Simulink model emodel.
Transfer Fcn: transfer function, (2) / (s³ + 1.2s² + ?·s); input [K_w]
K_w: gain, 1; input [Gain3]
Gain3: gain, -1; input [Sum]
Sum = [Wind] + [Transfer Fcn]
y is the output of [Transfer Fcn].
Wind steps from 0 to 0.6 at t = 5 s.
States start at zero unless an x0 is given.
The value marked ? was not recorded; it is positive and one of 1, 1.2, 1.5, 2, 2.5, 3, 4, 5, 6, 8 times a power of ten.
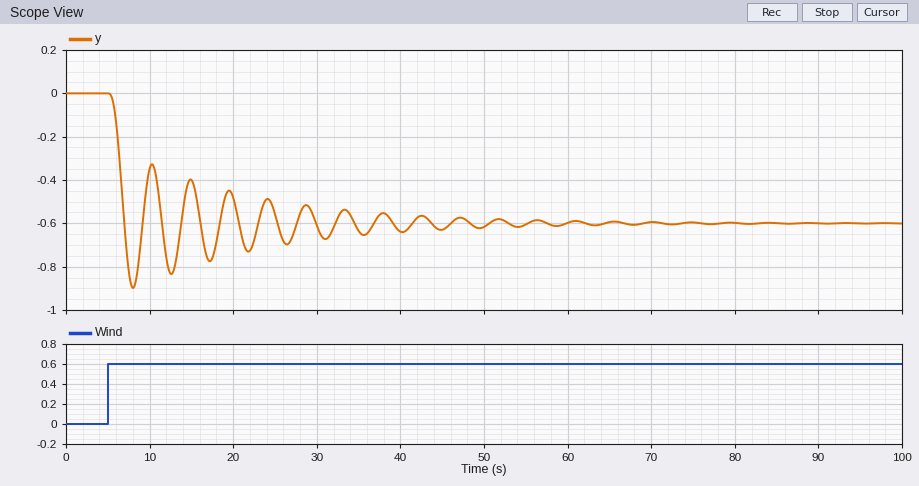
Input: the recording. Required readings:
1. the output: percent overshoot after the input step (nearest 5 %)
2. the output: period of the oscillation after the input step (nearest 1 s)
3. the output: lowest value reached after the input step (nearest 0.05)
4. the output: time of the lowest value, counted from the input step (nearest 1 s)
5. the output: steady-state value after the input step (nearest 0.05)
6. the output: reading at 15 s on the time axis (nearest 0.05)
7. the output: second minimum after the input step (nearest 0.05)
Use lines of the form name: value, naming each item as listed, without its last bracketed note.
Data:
the output: percent overshoot after the input step: 50 %
the output: period of the oscillation after the input step: 5 s
the output: lowest value reached after the input step: -0.90
the output: time of the lowest value, counted from the input step: 3 s
the output: steady-state value after the input step: -0.60
the output: reading at 15 s on the time axis: -0.40
the output: second minimum after the input step: -0.85
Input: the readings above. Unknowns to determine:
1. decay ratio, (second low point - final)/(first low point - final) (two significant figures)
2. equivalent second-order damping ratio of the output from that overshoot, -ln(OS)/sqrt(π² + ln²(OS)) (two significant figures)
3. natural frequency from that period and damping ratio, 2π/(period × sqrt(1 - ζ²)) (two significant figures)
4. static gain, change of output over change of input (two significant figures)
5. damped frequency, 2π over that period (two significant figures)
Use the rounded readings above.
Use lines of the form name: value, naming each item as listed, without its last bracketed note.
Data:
decay ratio, (second low point - final)/(first low point - final): 0.83
equivalent second-order damping ratio of the output from that overshoot, -ln(OS)/sqrt(π² + ln²(OS)): 0.22
natural frequency from that period and damping ratio, 2π/(period × sqrt(1 - ζ²)): 1.3 rad/s
static gain, change of output over change of input: -1.0
damped frequency, 2π over that period: 1.3 rad/s
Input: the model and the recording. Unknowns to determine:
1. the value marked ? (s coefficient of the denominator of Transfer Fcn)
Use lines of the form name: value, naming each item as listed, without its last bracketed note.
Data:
the value marked ?: 2
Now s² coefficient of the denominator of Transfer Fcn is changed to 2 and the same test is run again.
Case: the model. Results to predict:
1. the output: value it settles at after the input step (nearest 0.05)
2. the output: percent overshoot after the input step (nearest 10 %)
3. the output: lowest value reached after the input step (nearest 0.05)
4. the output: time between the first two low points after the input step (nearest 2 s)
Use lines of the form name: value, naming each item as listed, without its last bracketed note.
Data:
the output: value it settles at after the input step: -0.60
the output: percent overshoot after the input step: 40 %
the output: lowest value reached after the input step: -0.85
the output: time between the first two low points after the input step: 6 s
